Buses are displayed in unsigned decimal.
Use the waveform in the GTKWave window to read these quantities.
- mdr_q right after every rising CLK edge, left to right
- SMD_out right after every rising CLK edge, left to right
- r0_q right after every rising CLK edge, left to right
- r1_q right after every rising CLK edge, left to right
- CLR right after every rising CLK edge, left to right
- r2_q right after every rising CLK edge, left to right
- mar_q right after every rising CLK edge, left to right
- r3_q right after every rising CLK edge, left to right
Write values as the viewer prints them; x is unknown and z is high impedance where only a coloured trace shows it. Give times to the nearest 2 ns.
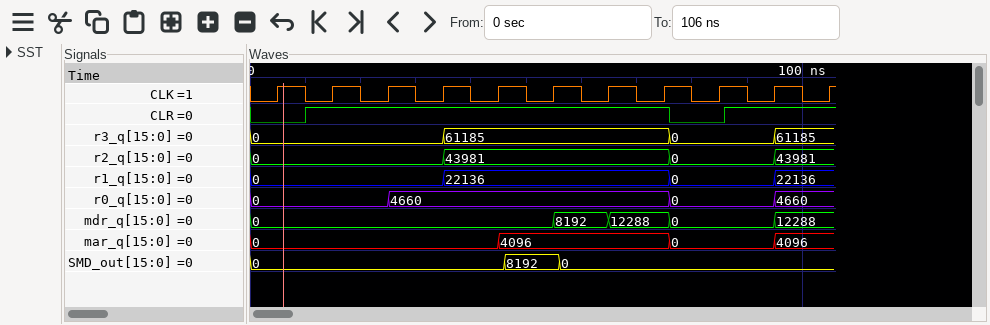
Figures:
0, 0, 0, 0, 0, 8192, 12288, 12288, 0, 12288, 12288
0, 0, 0, 0, 0, 8192, 0, 0, 0, 0, 0
0, 0, 4660, 4660, 4660, 4660, 4660, 4660, 0, 4660, 4660
0, 0, 0, 22136, 22136, 22136, 22136, 22136, 0, 22136, 22136
0 1 1 1 1 1 1 1 0 1 1
0, 0, 0, 43981, 43981, 43981, 43981, 43981, 0, 43981, 43981
0, 0, 0, 0, 4096, 4096, 4096, 4096, 0, 4096, 4096
0, 0, 0, 61185, 61185, 61185, 61185, 61185, 0, 61185, 61185
